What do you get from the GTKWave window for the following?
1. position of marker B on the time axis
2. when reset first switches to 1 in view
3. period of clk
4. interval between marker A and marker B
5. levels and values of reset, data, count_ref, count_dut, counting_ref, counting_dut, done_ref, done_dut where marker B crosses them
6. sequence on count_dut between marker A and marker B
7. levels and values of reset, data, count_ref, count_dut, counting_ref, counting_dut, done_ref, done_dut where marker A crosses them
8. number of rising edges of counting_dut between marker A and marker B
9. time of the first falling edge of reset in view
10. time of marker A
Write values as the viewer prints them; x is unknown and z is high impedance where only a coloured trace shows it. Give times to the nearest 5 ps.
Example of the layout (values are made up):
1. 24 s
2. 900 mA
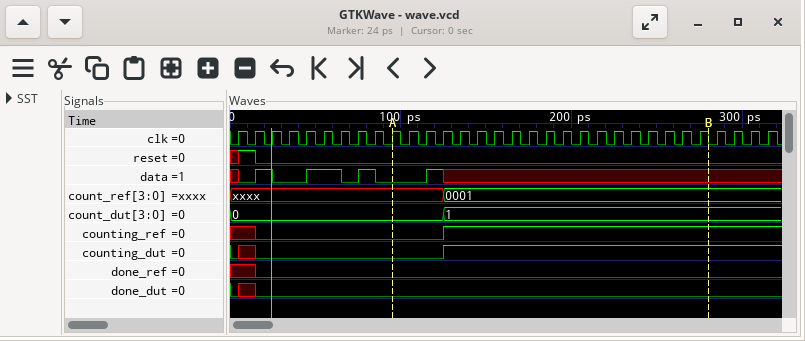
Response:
1. 280 ps
2. 5 ps
3. 10 ps
4. 185 ps
5. reset=0, data=x, count_ref=0001, count_dut=1, counting_ref=1, counting_dut=1, done_ref=0, done_dut=0
6. 0, 1
7. reset=0, data=0, count_ref=xxxx, count_dut=0, counting_ref=0, counting_dut=0, done_ref=0, done_dut=0
8. 1
9. 15 ps
10. 95 ps
